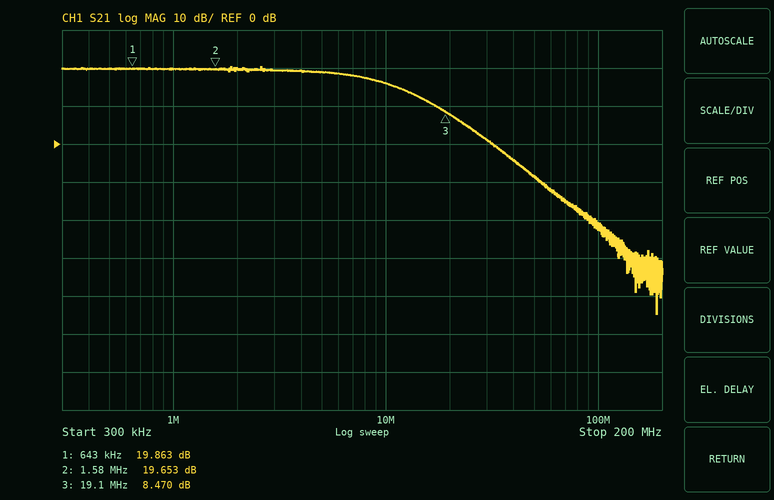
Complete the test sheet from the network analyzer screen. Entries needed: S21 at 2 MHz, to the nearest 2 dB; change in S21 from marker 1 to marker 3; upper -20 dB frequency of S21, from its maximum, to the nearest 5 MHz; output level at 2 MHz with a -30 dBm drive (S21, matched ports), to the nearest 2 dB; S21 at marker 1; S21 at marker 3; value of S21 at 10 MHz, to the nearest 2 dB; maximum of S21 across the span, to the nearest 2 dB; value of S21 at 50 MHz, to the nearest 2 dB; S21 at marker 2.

20 dB
-11.393 dB
30 MHz
-10 dBm
19.863 dB
8.470 dB
16 dB
20 dB
-8 dB
19.653 dB
